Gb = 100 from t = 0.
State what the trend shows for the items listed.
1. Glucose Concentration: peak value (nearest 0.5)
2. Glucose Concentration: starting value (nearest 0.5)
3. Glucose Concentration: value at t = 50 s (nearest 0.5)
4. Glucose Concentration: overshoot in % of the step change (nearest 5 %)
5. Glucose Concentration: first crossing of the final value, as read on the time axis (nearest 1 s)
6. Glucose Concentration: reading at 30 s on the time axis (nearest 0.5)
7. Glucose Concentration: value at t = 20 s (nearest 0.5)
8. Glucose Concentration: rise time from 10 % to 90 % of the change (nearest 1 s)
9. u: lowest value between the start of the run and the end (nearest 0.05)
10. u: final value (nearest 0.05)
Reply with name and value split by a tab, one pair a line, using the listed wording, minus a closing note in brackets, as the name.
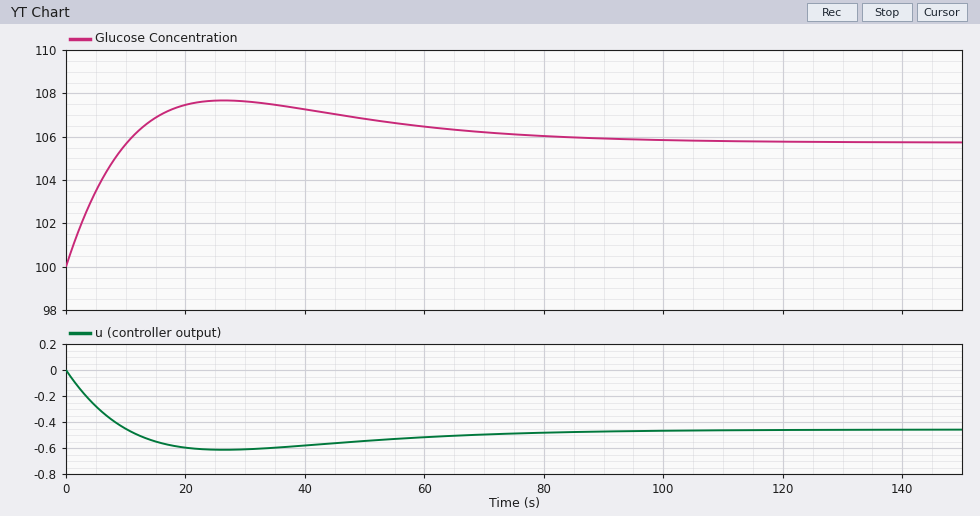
Glucose Concentration: peak value	107.5
Glucose Concentration: starting value	100.0
Glucose Concentration: value at t = 50 s	107.0
Glucose Concentration: overshoot in % of the step change	35 %
Glucose Concentration: first crossing of the final value, as read on the time axis	10 s
Glucose Concentration: reading at 30 s on the time axis	107.5
Glucose Concentration: value at t = 20 s	107.5
Glucose Concentration: rise time from 10 % to 90 % of the change	8 s
u: lowest value between the start of the run and the end	-0.60
u: final value	-0.45
